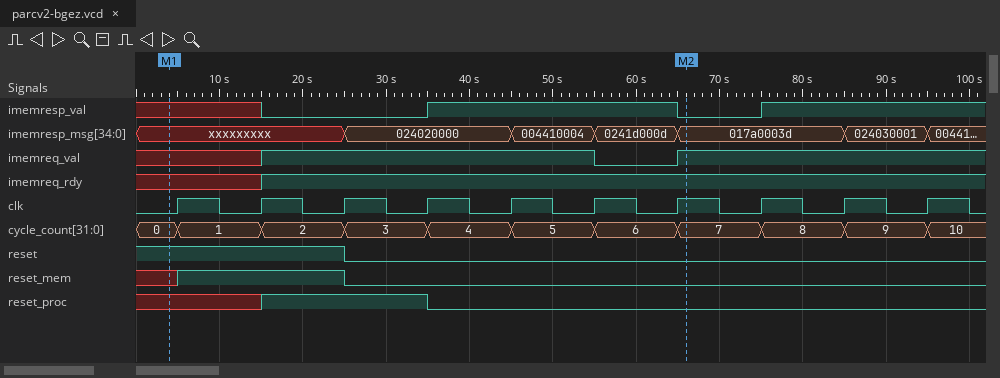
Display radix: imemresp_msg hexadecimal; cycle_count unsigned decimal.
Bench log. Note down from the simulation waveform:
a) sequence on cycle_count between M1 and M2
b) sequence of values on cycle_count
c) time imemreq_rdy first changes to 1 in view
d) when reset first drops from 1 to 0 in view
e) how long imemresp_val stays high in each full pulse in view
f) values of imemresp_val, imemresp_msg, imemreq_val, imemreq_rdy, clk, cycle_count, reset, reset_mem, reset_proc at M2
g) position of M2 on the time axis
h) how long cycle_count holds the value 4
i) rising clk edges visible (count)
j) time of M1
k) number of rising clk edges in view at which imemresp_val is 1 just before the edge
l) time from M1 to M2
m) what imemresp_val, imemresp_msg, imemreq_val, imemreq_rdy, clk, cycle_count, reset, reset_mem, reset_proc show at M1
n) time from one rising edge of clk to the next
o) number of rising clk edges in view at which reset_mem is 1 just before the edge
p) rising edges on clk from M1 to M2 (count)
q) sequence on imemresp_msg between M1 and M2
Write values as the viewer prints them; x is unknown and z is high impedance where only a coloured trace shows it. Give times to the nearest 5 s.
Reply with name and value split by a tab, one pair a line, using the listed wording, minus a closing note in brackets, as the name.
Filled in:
sequence on cycle_count between M1 and M2	0, 1, 2, 3, 4, 5, 6, 7
sequence of values on cycle_count	0, 1, 2, 3, 4, 5, 6, 7, 8, 9, 10
time imemreq_rdy first changes to 1 in view	15 s
when reset first drops from 1 to 0 in view	25 s
how long imemresp_val stays high in each full pulse in view	30 s
values of imemresp_val, imemresp_msg, imemreq_val, imemreq_rdy, clk, cycle_count, reset, reset_mem, reset_proc at M2	imemresp_val=0, imemresp_msg=017a0003d, imemreq_val=1, imemreq_rdy=1, clk=1, cycle_count=7, reset=0, reset_mem=0, reset_proc=0
position of M2 on the time axis	65 s
how long cycle_count holds the value 4	10 s
rising clk edges visible	10
time of M1	5 s
number of rising clk edges in view at which imemresp_val is 1 just before the edge	5
time from M1 to M2	60 s
what imemresp_val, imemresp_msg, imemreq_val, imemreq_rdy, clk, cycle_count, reset, reset_mem, reset_proc show at M1	imemresp_val=x, imemresp_msg=xxxxxxxxx, imemreq_val=x, imemreq_rdy=x, clk=0, cycle_count=0, reset=1, reset_mem=x, reset_proc=x
time from one rising edge of clk to the next	10 s
number of rising clk edges in view at which reset_mem is 1 just before the edge	2
rising edges on clk from M1 to M2	7
sequence on imemresp_msg between M1 and M2	xxxxxxxxx, 024020000, 004410004, 0241d000d, 017a0003d
